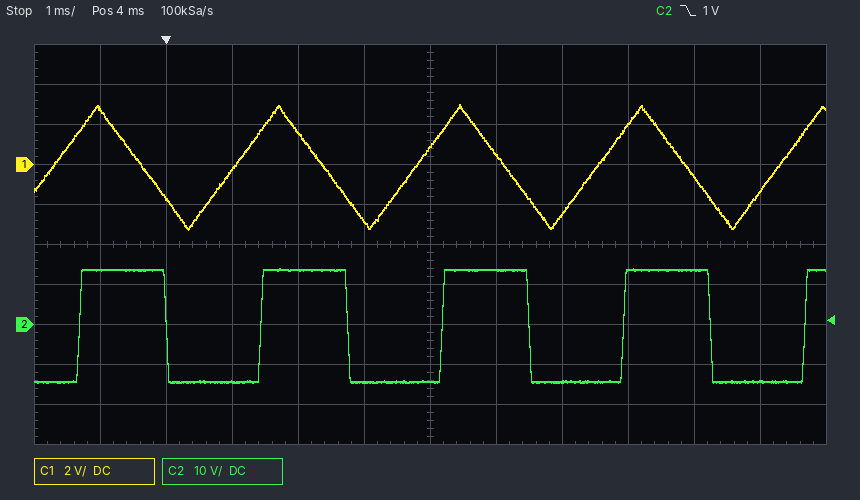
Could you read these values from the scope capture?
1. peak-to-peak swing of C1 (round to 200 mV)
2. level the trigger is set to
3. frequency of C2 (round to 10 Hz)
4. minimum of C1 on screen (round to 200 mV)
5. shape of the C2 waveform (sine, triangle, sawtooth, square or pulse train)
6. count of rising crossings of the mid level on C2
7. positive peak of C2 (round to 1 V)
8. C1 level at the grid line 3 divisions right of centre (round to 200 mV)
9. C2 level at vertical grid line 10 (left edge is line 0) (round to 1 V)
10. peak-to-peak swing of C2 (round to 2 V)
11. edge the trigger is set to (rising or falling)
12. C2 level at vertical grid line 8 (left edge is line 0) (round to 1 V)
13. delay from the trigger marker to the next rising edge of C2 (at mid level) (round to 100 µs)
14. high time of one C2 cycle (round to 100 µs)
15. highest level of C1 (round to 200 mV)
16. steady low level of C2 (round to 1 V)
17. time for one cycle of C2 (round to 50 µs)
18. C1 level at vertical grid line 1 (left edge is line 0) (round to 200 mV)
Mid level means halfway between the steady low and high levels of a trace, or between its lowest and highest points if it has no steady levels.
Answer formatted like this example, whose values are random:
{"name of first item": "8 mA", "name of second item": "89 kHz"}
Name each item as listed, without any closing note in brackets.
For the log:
{"peak-to-peak swing of C1": "6.2 V", "level the trigger is set to": "1 V", "frequency of C2": "360 Hz", "minimum of C1 on screen": "-3.2 V", "shape of the C2 waveform": "square", "count of rising crossings of the mid level on C2": "5", "positive peak of C2": "14 V", "C1 level at the grid line 3 divisions right of centre": "2.0 V", "C2 level at vertical grid line 10 (left edge is line 0)": "14 V", "peak-to-peak swing of C2": "28 V", "edge the trigger is set to": "falling", "C2 level at vertical grid line 8 (left edge is line 0)": "-14 V", "delay from the trigger marker to the next rising edge of C2 (at mid level)": "1.4 ms", "high time of one C2 cycle": "1.3 ms", "highest level of C1": "3.0 V", "steady low level of C2": "-14 V", "time for one cycle of C2": "2.75 ms", "C1 level at vertical grid line 1 (left edge is line 0)": "2.8 V"}
